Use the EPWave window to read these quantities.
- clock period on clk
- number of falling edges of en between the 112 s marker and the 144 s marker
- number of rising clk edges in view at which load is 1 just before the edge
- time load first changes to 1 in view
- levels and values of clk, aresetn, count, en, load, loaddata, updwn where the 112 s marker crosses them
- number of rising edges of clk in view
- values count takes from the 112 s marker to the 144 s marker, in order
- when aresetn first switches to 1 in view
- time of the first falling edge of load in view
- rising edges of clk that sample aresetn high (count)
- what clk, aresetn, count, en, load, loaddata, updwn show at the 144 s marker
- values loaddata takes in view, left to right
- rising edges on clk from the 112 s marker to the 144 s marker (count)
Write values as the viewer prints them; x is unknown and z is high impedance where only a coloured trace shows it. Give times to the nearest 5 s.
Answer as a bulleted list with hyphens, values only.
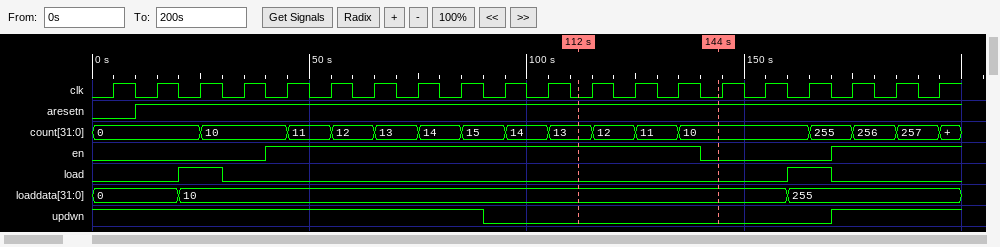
- 10 s
- 1
- 2
- 20 s
- clk=0, aresetn=1, count=13, en=1, load=0, loaddata=10, updwn=0
- 20
- 13, 12, 11, 10
- 10 s
- 30 s
- 19
- clk=0, aresetn=1, count=10, en=0, load=0, loaddata=10, updwn=0
- 0, 10, 255
- 3
